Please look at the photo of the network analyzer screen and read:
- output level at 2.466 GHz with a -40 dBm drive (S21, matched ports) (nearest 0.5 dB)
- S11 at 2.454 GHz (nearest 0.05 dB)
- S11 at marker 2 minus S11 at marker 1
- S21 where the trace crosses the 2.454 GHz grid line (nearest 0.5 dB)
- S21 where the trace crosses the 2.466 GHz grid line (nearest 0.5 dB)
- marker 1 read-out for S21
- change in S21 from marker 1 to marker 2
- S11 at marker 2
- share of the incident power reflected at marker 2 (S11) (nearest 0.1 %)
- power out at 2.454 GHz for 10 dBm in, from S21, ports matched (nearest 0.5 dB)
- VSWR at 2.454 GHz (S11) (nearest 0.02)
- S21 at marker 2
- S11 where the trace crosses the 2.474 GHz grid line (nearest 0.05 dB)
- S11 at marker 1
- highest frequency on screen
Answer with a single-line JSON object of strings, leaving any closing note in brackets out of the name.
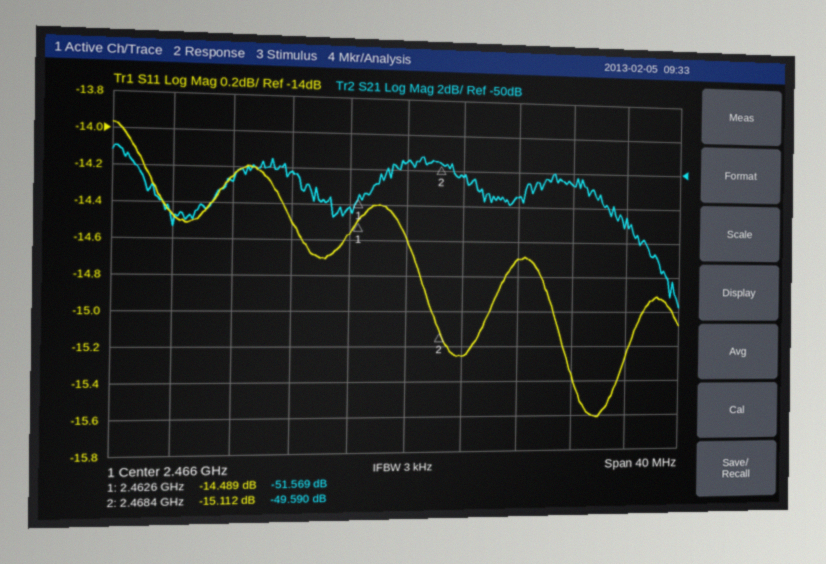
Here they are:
{"output level at 2.466 GHz with a -40 dBm drive (S21, matched ports)": "-89.5 dBm", "S11 at 2.454 GHz": "-14.25 dB", "S11 at marker 2 minus S11 at marker 1": "-0.623 dB", "S21 where the trace crosses the 2.454 GHz grid line": "-51.0 dB", "S21 where the trace crosses the 2.466 GHz grid line": "-49.5 dB", "marker 1 read-out for S21": "-51.569 dB", "change in S21 from marker 1 to marker 2": "1.979 dB", "S11 at marker 2": "-15.112 dB", "share of the incident power reflected at marker 2 (S11)": "3.1 %", "power out at 2.454 GHz for 10 dBm in, from S21, ports matched": "-41.0 dBm", "VSWR at 2.454 GHz (S11)": "1.48", "S21 at marker 2": "-49.590 dB", "S11 where the trace crosses the 2.474 GHz grid line": "-14.70 dB", "S11 at marker 1": "-14.489 dB", "highest frequency on screen": "2.486 GHz"}
